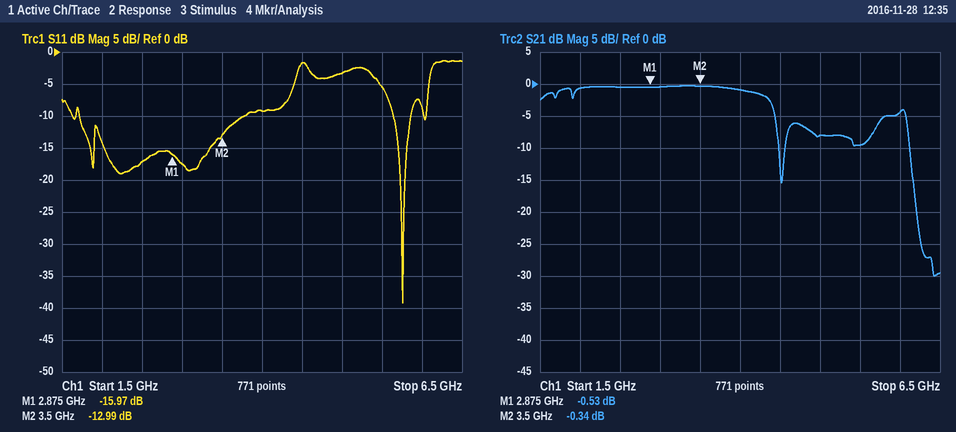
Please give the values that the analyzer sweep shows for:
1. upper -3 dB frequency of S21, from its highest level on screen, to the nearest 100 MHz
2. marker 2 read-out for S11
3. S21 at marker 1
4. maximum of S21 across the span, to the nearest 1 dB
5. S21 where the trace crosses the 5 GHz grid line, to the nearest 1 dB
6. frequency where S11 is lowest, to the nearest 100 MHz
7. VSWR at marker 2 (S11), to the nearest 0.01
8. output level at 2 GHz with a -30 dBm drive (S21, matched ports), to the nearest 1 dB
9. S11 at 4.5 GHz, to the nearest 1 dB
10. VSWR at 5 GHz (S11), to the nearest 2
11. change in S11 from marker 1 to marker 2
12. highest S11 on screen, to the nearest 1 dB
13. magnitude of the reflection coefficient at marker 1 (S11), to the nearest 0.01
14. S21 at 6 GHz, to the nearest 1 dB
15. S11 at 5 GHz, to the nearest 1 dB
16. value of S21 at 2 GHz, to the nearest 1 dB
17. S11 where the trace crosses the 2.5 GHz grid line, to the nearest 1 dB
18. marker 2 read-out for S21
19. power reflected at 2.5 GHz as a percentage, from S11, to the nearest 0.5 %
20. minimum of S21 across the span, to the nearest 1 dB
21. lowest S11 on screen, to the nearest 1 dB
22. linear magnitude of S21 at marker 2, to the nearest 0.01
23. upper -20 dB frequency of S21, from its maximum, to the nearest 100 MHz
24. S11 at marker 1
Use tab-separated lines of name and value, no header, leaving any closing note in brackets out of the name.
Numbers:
upper -3 dB frequency of S21, from its highest level on screen, to the nearest 100 MHz	4.4 GHz
marker 2 read-out for S11	-12.99 dB
S21 at marker 1	-0.53 dB
maximum of S21 across the span, to the nearest 1 dB	0 dB
S21 where the trace crosses the 5 GHz grid line, to the nearest 1 dB	-8 dB
frequency where S11 is lowest, to the nearest 100 MHz	5.8 GHz
VSWR at marker 2 (S11), to the nearest 0.01	1.58
output level at 2 GHz with a -30 dBm drive (S21, matched ports), to the nearest 1 dB	-31 dBm
S11 at 4.5 GHz, to the nearest 1 dB	-2 dB
VSWR at 5 GHz (S11), to the nearest 2	6
change in S11 from marker 1 to marker 2	2.98 dB
highest S11 on screen, to the nearest 1 dB	-1 dB
magnitude of the reflection coefficient at marker 1 (S11), to the nearest 0.01	0.16
S21 at 6 GHz, to the nearest 1 dB	-4 dB
S11 at 5 GHz, to the nearest 1 dB	-3 dB
value of S21 at 2 GHz, to the nearest 1 dB	-1 dB
S11 where the trace crosses the 2.5 GHz grid line, to the nearest 1 dB	-17 dB
marker 2 read-out for S21	-0.34 dB
power reflected at 2.5 GHz as a percentage, from S11, to the nearest 0.5 %	2.0 %
minimum of S21 across the span, to the nearest 1 dB	-30 dB
lowest S11 on screen, to the nearest 1 dB	-39 dB
linear magnitude of S21 at marker 2, to the nearest 0.01	0.96
upper -20 dB frequency of S21, from its maximum, to the nearest 100 MHz	6.2 GHz
S11 at marker 1	-15.97 dB
